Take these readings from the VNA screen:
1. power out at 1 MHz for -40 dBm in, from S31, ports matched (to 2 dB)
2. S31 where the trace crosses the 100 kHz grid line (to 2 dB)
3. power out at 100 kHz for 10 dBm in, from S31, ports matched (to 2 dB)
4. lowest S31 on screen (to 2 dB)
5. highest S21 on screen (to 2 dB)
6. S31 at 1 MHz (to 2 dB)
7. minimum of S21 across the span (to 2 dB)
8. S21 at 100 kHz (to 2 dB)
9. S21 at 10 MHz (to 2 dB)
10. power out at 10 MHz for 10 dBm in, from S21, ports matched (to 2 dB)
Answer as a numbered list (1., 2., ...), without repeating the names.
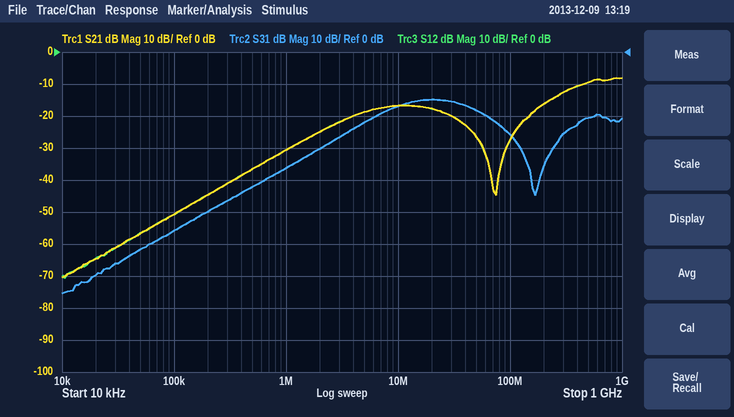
1. -76 dBm
2. -56 dB
3. -46 dBm
4. -76 dB
5. -8 dB
6. -36 dB
7. -70 dB
8. -50 dB
9. -16 dB
10. -6 dBm
